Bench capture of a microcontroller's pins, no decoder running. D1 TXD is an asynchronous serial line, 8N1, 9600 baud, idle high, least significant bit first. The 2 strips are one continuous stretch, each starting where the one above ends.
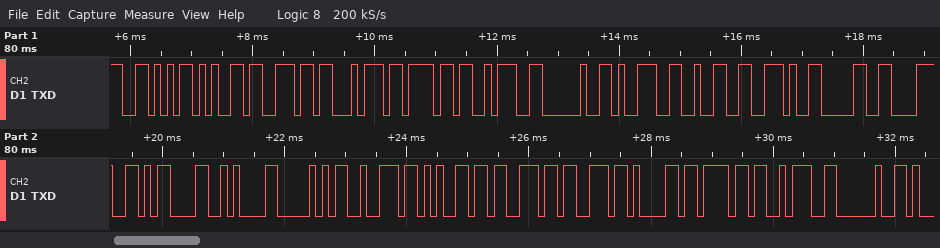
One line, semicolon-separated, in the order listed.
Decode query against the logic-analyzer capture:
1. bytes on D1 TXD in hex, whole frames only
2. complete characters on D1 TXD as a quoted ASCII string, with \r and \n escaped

0x56 0x65 0x6E 0x74 0x6F 0x3A 0x20 0x39 0x32 0x2E 0x30 0x38 0x0D 0x0A 0x50 0x72 0x65 0x73 0x73 0x61 0x6F 0x3A 0x20; "Vento: 92.08\r\nPressao: "
